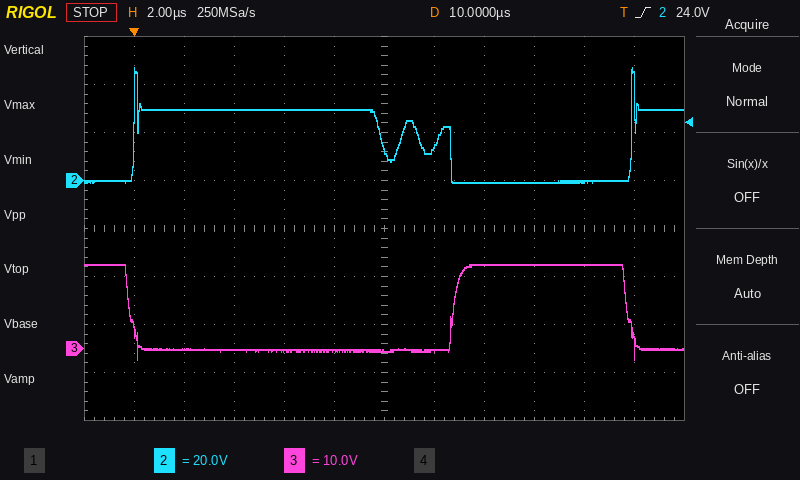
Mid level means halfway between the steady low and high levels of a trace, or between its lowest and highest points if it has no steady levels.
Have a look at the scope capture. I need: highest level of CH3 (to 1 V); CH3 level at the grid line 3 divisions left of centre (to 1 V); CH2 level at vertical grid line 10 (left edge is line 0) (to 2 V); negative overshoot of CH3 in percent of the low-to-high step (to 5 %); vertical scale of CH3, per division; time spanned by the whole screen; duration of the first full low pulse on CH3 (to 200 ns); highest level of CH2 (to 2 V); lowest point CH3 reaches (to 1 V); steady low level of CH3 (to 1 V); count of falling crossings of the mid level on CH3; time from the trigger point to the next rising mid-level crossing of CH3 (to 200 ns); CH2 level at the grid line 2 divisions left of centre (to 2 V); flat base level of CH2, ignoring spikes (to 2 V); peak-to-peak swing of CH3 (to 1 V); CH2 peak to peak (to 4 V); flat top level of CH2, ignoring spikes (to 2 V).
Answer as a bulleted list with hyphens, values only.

- 18 V
- 0 V
- 0 V
- 10 %
- 10 V
- 24 µs
- 13.0 µs
- 48 V
- -2 V
- 0 V
- 2
- 12.8 µs
- 30 V
- 0 V
- 20 V
- 48 V
- 30 V
